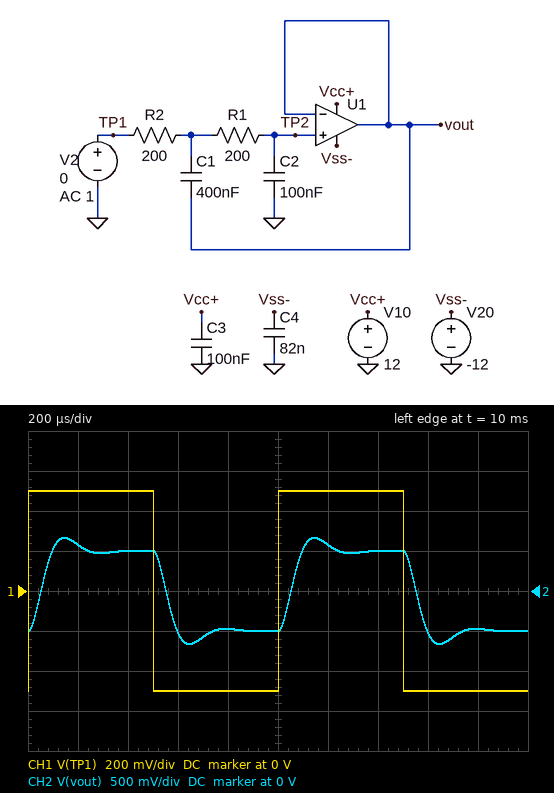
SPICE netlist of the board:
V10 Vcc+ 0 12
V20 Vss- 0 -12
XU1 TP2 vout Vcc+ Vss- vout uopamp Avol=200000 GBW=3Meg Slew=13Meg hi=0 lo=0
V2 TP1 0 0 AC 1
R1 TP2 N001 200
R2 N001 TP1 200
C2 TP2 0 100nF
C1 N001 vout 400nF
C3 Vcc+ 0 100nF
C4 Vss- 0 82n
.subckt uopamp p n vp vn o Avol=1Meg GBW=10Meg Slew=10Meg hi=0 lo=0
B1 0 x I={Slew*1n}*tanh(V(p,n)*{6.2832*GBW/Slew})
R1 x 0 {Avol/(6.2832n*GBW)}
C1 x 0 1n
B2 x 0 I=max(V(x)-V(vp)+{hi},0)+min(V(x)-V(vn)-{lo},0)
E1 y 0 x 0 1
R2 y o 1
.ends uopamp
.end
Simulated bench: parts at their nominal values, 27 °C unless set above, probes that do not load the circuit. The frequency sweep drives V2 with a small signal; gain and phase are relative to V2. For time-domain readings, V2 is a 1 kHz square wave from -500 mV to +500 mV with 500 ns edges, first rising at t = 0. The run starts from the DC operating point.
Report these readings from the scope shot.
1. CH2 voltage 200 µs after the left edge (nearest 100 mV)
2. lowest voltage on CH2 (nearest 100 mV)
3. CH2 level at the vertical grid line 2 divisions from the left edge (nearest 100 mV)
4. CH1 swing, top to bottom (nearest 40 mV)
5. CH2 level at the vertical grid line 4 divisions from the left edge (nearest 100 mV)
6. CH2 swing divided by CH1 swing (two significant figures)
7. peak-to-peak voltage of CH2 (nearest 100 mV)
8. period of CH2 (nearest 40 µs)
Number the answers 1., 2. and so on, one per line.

1. 600 mV
2. -700 mV
3. 500 mV
4. 1.00 V
5. -500 mV
6. 1.3
7. 1.3 V
8. 1.00 ms
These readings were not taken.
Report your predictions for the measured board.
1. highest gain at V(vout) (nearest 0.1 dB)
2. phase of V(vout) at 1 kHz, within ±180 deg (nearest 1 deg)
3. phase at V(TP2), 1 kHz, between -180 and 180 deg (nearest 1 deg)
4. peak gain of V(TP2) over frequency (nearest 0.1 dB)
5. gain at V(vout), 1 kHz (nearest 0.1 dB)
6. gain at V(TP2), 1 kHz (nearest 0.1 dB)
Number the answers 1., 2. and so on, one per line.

1. 1.3 dB
2. -15 deg
3. -15 deg
4. 1.3 dB
5. 0.3 dB
6. 0.3 dB
